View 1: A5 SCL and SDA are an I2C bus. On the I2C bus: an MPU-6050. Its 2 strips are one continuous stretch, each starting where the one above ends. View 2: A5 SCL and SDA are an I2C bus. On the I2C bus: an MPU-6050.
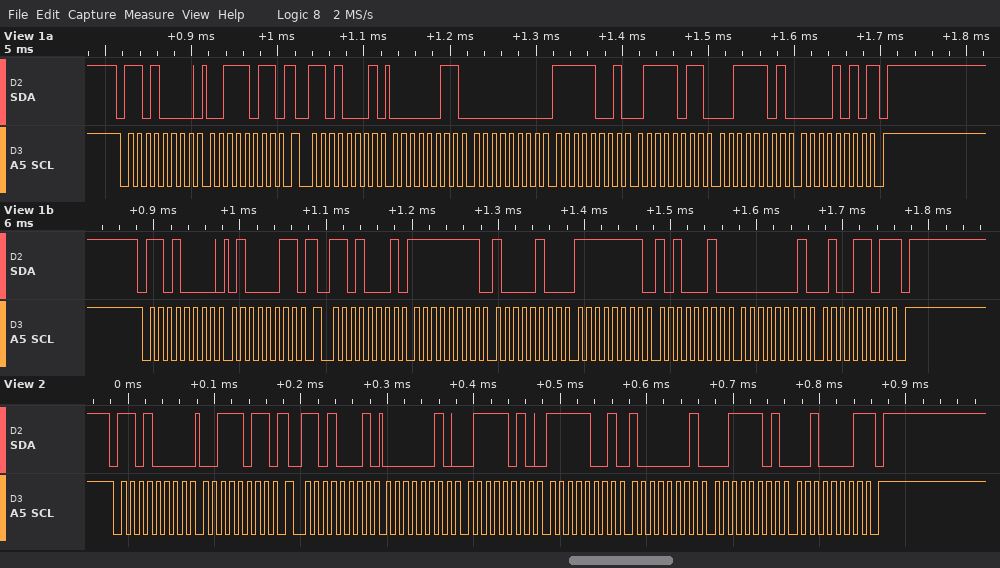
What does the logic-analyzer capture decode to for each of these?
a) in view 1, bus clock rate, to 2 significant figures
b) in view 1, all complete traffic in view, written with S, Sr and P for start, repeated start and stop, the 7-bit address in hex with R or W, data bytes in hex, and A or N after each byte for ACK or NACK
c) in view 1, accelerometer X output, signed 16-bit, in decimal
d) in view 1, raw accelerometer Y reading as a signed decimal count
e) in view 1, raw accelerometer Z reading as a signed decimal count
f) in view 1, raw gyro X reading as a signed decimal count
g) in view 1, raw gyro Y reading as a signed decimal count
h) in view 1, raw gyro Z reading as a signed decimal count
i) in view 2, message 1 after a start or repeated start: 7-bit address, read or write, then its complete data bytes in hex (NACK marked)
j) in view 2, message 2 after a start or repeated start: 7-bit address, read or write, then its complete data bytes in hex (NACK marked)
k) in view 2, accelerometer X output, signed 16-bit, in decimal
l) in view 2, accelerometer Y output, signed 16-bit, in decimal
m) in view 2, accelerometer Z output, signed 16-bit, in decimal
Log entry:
100 kHz
S 68W A 3B A Sr 68R A 03 A 00 A F9 A 7B A 3D A 0A N P S 68W A 43 A Sr 68R A FF A 84 A FF A A2 A 01 A 4D N P
768
-1669
15626
-124
-94
333
0x68 write: 3B
0x68 read: 02 7A F9 81 3D 21 NACK
634
-1663
15649
